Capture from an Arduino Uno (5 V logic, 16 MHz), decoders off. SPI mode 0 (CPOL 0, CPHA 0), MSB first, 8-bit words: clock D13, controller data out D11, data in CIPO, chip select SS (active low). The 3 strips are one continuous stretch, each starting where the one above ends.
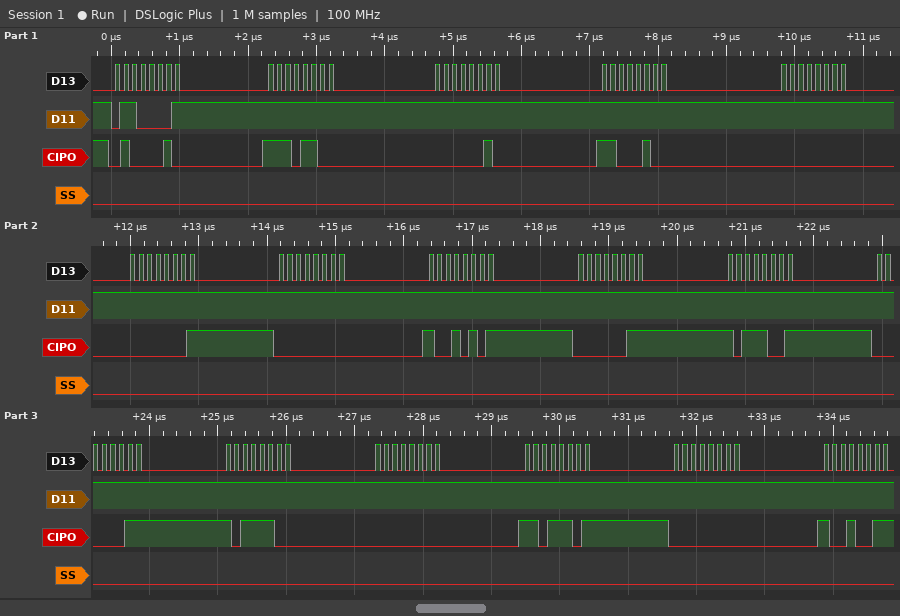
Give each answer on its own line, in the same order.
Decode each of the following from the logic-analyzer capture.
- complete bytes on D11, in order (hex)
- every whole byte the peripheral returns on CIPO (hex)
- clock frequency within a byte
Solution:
0x61 0xFF 0xFF 0xFF 0xFF 0xFF 0xFF 0xFF 0xFF 0xFF 0xFF 0xFF 0xFF 0xFF 0xFF 0xFF
0x42 0xEC 0x02 0xC4 0x00 0x01 0x00 0x95 0x03 0xB9 0x03 0xBC 0x00 0xDD 0x00 0x93
8 MHz
